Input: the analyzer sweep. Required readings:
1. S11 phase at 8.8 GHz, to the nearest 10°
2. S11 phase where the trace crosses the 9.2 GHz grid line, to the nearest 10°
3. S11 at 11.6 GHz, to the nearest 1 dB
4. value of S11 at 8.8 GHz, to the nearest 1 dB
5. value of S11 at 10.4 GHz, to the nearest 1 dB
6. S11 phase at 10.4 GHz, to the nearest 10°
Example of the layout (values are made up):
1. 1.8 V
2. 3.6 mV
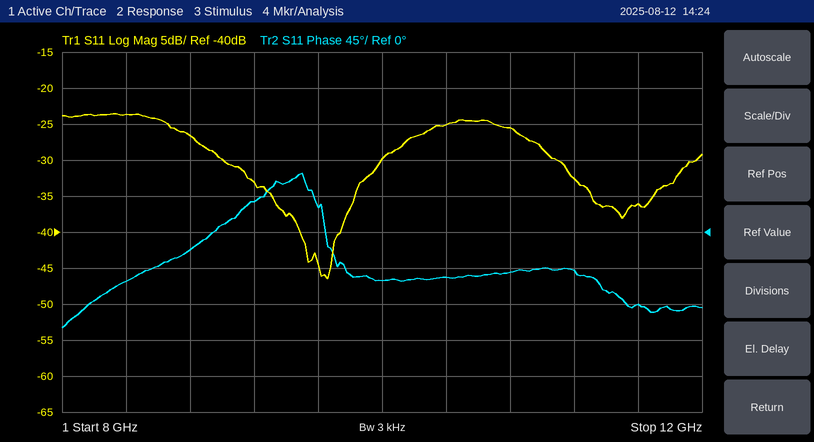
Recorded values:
1. -20°
2. 40°
3. -36 dB
4. -27 dB
5. -25 dB
6. -60°
